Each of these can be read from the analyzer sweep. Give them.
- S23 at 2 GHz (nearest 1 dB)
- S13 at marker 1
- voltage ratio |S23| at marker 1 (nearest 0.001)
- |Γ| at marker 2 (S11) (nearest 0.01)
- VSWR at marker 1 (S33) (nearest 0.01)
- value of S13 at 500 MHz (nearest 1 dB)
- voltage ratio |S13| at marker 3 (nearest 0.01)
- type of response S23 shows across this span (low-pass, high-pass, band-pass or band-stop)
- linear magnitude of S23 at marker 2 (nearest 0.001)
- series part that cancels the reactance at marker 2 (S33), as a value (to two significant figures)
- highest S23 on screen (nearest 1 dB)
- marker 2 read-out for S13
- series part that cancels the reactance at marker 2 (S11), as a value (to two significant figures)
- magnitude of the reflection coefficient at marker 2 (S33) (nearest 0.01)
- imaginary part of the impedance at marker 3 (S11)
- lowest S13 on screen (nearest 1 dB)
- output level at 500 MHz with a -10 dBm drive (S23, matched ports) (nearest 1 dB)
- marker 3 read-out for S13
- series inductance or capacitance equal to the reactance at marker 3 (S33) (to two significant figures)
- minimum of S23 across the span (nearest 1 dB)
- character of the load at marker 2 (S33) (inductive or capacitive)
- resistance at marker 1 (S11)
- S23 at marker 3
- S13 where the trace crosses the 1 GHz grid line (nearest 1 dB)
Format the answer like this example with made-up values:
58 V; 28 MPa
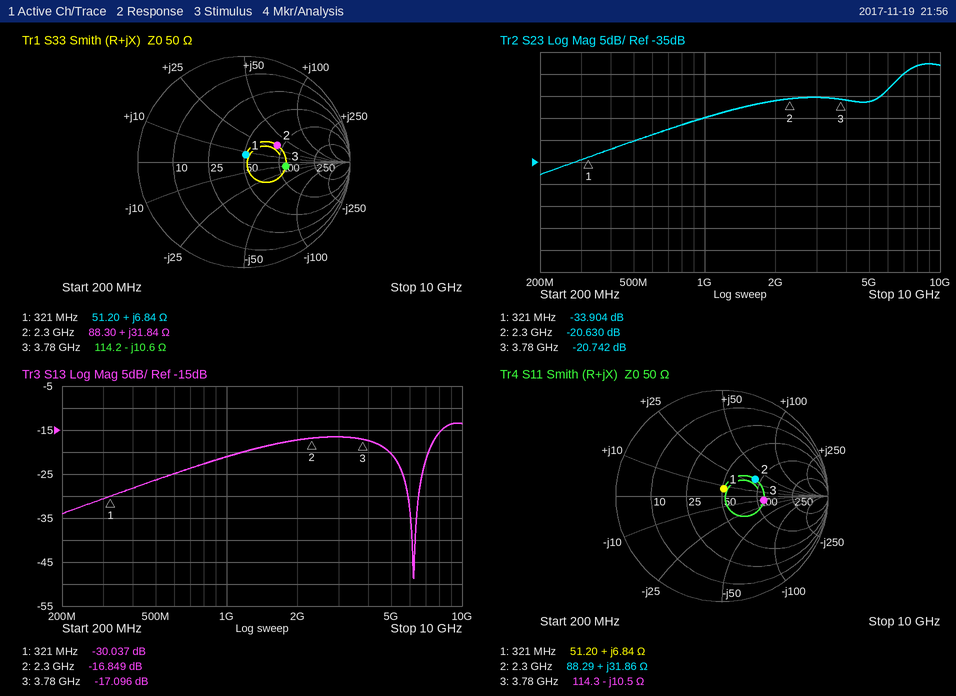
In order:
-21 dB; -30.037 dB; 0.020; 0.35; 1.15; -26 dB; 0.14; high-pass; 0.093; 2.2 pF; -13 dB; -16.849 dB; 2.2 pF; 0.35; -10.5 Ω; -49 dB; -40 dBm; -17.096 dB; 4.0 pF; -38 dB; inductive; 51.20 Ω; -20.742 dB; -21 dB
